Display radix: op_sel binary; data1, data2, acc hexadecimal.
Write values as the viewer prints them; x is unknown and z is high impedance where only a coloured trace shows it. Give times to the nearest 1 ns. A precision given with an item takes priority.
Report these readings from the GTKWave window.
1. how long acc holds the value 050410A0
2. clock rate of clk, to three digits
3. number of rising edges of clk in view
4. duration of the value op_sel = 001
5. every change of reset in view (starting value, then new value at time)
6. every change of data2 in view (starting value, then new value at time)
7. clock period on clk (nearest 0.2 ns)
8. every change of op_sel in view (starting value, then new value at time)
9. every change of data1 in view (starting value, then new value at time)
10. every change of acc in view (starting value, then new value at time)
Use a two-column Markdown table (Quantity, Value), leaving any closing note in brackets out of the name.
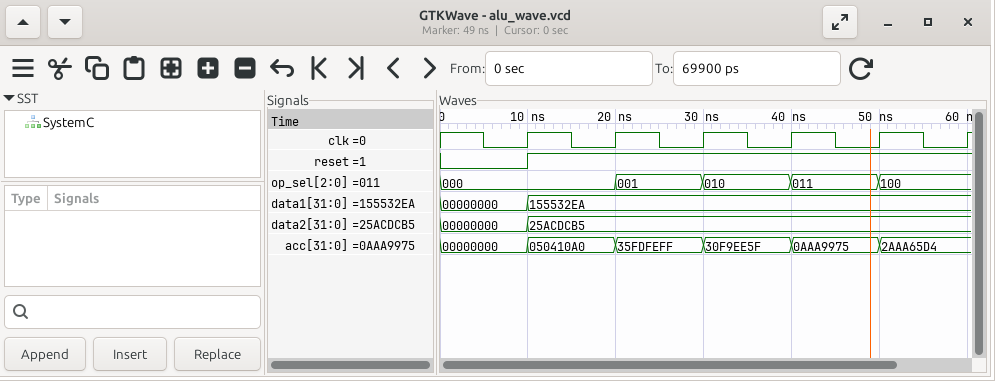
| Quantity | Value |
|---|---|
| how long acc holds the value 050410A0 | 10 ns |
| clock rate of clk, to three digits | 100 MHz |
| number of rising edges of clk in view | 6 |
| duration of the value op_sel = 001 | 10 ns |
| every change of reset in view | 0, 1 at 10 ns |
| every change of data2 in view | 00000000, 25ACDCB5 at 10 ns |
| clock period on clk | 10 ns |
| every change of op_sel in view | 000, 001 at 20 ns, 010 at 30 ns, 011 at 40 ns, 100 at 50 ns |
| every change of data1 in view | 00000000, 155532EA at 10 ns |
| every change of acc in view | 00000000, 050410A0 at 10 ns, 35FDFEFF at 20 ns, 30F9EE5F at 30 ns, 0AAA9975 at 40 ns, 2AAA65D4 at 50 ns |
